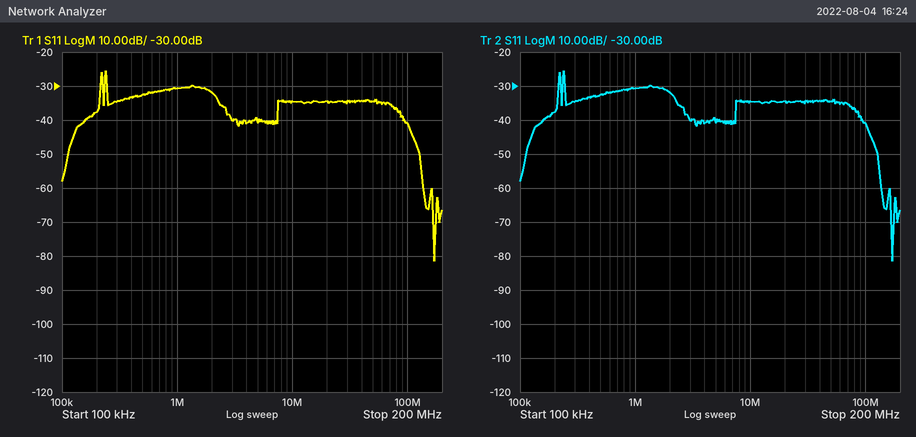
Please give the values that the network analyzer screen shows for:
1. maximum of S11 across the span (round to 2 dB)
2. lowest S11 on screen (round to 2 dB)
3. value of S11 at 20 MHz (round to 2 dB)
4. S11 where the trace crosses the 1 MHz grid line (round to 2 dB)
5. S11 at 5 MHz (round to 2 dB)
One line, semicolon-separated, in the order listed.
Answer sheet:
-26 dB; -82 dB; -34 dB; -30 dB; -40 dB
